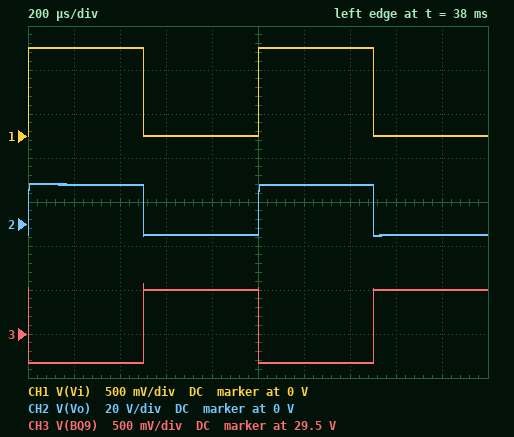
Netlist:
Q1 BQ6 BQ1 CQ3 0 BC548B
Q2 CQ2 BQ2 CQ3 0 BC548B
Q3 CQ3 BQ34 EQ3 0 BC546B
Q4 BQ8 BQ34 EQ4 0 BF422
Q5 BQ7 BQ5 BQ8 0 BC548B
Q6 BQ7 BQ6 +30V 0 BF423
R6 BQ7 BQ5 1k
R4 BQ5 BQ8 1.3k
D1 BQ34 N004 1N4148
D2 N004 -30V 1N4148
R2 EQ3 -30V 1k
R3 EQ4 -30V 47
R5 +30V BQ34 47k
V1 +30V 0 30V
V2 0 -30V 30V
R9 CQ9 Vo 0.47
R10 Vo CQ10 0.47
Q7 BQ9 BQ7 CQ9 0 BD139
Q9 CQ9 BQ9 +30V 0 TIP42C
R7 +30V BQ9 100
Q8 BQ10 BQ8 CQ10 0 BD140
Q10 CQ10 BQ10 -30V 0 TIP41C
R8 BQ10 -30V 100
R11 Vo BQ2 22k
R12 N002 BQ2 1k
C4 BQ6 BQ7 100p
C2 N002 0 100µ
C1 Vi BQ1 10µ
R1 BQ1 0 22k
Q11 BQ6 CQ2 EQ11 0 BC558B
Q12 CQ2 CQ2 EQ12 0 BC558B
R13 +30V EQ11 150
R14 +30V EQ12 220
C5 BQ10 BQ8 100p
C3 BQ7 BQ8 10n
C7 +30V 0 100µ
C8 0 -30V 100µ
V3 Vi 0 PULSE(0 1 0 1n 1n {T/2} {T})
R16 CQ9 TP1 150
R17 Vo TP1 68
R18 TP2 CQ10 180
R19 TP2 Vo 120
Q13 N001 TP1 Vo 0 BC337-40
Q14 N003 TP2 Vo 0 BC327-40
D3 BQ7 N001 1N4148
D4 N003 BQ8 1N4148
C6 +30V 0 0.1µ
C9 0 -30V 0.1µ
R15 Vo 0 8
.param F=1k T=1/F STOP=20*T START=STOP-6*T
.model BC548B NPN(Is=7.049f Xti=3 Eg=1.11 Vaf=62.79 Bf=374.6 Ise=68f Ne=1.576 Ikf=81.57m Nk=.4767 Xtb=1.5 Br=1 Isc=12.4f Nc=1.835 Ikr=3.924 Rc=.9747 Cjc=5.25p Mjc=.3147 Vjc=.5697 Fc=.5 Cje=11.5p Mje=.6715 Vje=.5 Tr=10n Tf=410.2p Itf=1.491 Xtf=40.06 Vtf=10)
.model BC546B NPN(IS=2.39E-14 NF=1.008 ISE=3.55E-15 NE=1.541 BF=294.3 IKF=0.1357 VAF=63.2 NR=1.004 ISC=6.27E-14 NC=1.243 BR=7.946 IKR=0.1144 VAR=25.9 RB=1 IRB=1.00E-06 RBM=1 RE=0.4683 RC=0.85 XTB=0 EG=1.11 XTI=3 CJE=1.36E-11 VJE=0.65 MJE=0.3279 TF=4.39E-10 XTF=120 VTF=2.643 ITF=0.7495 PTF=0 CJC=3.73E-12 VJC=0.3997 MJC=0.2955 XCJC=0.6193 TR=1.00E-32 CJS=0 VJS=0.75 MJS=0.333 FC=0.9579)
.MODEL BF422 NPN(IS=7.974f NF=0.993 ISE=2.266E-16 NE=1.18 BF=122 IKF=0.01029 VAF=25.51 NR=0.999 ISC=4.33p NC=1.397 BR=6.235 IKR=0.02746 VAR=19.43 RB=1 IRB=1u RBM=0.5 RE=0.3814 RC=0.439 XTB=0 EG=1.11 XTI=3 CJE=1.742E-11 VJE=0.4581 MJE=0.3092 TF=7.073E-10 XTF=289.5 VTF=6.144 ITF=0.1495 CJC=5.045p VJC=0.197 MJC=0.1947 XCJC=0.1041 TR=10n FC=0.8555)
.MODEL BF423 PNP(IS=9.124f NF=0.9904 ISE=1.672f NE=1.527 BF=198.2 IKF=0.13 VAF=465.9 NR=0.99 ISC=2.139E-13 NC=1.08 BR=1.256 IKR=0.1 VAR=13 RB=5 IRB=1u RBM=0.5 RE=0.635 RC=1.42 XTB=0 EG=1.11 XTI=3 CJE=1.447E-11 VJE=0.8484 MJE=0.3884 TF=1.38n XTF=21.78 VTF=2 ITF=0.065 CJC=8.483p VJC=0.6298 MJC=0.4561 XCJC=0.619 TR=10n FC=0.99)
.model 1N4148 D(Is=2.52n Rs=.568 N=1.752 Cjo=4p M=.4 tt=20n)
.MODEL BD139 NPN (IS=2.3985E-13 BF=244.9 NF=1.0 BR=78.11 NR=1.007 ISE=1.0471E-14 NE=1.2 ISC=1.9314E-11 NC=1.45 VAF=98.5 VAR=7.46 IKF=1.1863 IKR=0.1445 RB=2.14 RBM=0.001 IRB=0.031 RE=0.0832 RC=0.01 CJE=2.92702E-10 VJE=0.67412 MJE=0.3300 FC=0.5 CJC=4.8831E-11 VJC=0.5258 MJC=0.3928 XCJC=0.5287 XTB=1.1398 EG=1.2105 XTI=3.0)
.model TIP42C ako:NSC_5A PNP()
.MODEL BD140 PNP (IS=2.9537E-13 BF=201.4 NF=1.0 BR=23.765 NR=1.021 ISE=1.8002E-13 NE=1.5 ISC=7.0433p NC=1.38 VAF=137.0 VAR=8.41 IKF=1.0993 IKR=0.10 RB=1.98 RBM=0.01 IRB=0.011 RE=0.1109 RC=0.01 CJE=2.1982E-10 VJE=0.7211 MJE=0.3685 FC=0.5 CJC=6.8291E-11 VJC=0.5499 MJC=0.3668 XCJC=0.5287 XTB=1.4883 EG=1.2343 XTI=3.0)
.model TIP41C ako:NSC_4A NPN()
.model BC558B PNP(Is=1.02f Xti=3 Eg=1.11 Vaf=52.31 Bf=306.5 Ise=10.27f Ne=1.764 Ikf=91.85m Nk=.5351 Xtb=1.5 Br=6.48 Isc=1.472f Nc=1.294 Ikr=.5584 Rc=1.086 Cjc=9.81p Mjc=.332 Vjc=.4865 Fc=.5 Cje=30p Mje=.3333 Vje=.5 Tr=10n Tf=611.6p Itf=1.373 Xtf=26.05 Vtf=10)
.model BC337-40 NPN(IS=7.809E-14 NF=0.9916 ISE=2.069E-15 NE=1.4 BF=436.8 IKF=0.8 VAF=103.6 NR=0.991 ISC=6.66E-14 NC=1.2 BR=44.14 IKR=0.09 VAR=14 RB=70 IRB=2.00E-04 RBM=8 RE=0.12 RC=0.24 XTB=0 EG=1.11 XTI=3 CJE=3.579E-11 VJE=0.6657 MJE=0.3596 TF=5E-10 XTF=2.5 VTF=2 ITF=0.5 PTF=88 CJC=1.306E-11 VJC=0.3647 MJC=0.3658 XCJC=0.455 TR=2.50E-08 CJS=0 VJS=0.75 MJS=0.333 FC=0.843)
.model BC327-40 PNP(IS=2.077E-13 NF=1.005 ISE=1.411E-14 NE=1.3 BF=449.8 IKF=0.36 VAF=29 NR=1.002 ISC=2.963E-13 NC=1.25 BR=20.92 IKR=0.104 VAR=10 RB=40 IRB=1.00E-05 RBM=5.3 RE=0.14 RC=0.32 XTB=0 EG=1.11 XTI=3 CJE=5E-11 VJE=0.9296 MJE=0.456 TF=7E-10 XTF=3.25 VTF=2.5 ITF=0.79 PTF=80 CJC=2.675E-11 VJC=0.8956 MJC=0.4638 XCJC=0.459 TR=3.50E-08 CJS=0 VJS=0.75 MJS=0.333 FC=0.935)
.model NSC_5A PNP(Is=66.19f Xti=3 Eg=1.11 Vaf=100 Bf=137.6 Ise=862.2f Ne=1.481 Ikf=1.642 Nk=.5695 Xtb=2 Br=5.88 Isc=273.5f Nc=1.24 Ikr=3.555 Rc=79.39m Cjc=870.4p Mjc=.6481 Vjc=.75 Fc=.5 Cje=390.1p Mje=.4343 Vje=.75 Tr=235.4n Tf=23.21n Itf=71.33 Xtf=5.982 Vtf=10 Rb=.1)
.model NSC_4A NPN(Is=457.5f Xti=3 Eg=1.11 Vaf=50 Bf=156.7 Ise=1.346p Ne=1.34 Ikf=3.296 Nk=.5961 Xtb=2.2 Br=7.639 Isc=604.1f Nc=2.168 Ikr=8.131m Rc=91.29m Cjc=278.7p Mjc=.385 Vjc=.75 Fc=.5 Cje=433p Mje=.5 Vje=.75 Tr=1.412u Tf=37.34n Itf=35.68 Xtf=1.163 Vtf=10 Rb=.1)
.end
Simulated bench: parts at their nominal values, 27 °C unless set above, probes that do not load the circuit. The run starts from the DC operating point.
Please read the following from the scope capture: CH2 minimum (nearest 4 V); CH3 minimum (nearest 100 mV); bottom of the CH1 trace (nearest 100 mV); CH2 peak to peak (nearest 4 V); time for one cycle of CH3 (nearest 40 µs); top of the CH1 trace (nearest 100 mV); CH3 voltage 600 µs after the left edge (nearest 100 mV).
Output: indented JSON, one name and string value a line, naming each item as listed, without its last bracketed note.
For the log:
{
  "CH2 minimum": "-4 V",
  "CH3 minimum": "29.2 V",
  "bottom of the CH1 trace": "0 V",
  "CH2 peak to peak": "24 V",
  "time for one cycle of CH3": "1.00 ms",
  "top of the CH1 trace": "1.0 V",
  "CH3 voltage 600 µs after the left edge": "30.0 V"
}
